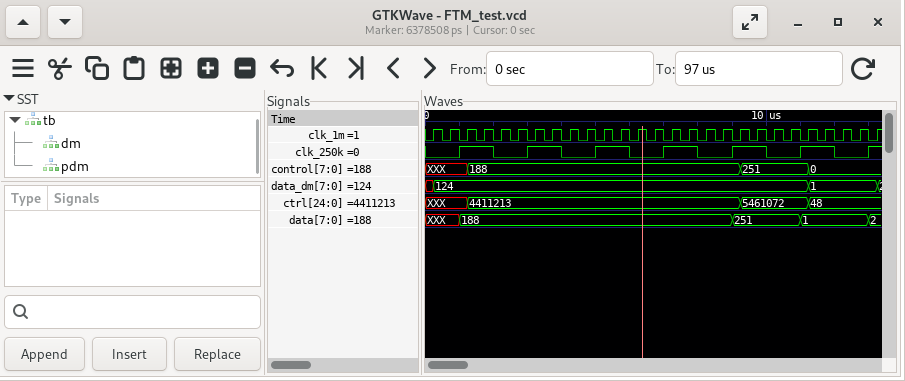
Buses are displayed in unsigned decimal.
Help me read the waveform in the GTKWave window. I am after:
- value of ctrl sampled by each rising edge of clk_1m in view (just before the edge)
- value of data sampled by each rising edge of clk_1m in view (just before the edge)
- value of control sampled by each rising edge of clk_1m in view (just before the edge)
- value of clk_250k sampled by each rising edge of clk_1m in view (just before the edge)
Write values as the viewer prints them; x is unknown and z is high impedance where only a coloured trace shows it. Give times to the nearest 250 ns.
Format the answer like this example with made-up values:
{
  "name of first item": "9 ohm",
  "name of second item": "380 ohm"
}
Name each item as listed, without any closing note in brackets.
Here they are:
{
  "value of ctrl sampled by each rising edge of clk_1m in view": "XXX, XXX, XXX, 4411213, 4411213, 4411213, 4411213, 4411213, 4411213, 4411213, 4411213, 4411213, 4411213, 4411213, 4411213, 4411213, 4411213, 4411213, 4411213, 5461072, 5461072, 5461072, 5461072, 48, 48, 48, 48",
  "value of data sampled by each rising edge of clk_1m in view": "XXX, XXX, 188, 188, 188, 188, 188, 188, 188, 188, 188, 188, 188, 188, 188, 188, 188, 188, 251, 251, 251, 251, 1, 1, 1, 1, 2",
  "value of control sampled by each rising edge of clk_1m in view": "XXX, XXX, XXX, 188, 188, 188, 188, 188, 188, 188, 188, 188, 188, 188, 188, 188, 188, 188, 188, 251, 251, 251, 251, 0, 0, 0, 0",
  "value of clk_250k sampled by each rising edge of clk_1m in view": "0 0 1 1 0 0 1 1 0 0 1 1 0 0 1 1 0 0 1 1 0 0 1 1 0 0 1"
}
